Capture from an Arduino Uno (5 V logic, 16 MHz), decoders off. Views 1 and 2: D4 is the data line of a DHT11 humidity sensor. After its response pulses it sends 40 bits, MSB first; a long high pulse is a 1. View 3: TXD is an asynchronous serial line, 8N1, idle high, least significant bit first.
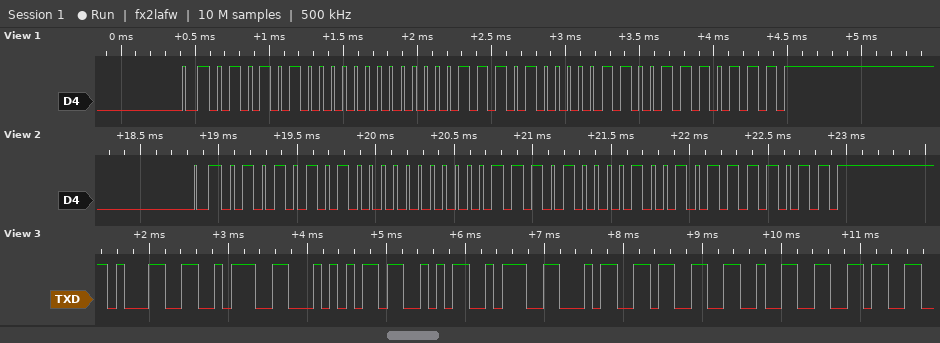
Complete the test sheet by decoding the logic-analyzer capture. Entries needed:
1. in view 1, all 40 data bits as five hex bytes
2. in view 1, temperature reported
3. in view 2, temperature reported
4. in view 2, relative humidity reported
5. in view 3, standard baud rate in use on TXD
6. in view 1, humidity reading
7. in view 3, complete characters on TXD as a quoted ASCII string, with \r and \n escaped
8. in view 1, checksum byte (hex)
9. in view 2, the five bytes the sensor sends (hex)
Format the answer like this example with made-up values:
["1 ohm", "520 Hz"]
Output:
["54 00 1D 06 77", "29.6 °C", "29.9 °C", "85 %", "9600 baud", "84 %", "\"1:TS:4326\"", "0x77", "55 00 1D 09 7B"]
